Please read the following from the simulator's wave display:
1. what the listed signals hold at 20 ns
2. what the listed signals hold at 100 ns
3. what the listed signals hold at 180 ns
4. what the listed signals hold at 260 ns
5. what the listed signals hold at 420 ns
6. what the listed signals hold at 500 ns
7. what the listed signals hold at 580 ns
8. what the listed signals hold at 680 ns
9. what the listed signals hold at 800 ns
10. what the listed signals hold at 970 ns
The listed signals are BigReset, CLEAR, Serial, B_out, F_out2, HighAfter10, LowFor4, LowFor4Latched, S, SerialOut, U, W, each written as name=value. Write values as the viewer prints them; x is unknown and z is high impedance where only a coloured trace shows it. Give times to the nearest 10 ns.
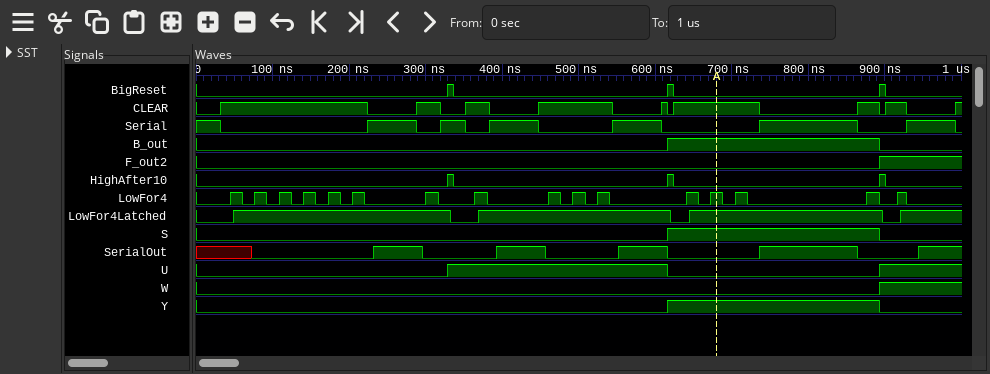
BigReset=0, CLEAR=0, Serial=1, B_out=0, F_out2=0, HighAfter10=0, LowFor4=0, LowFor4Latched=0, S=0, SerialOut=x, U=0, W=0
BigReset=0, CLEAR=1, Serial=0, B_out=0, F_out2=0, HighAfter10=0, LowFor4=0, LowFor4Latched=1, S=0, SerialOut=0, U=0, W=0
BigReset=0, CLEAR=1, Serial=0, B_out=0, F_out2=0, HighAfter10=0, LowFor4=1, LowFor4Latched=1, S=0, SerialOut=0, U=0, W=0
BigReset=0, CLEAR=0, Serial=1, B_out=0, F_out2=0, HighAfter10=0, LowFor4=0, LowFor4Latched=1, S=0, SerialOut=1, U=0, W=0
BigReset=0, CLEAR=0, Serial=1, B_out=0, F_out2=0, HighAfter10=0, LowFor4=0, LowFor4Latched=1, S=0, SerialOut=1, U=1, W=0
BigReset=0, CLEAR=1, Serial=0, B_out=0, F_out2=0, HighAfter10=0, LowFor4=1, LowFor4Latched=1, S=0, SerialOut=0, U=1, W=0
BigReset=0, CLEAR=0, Serial=1, B_out=0, F_out2=0, HighAfter10=0, LowFor4=0, LowFor4Latched=1, S=0, SerialOut=1, U=1, W=0
BigReset=0, CLEAR=1, Serial=0, B_out=1, F_out2=0, HighAfter10=0, LowFor4=1, LowFor4Latched=1, S=1, SerialOut=0, U=0, W=0
BigReset=0, CLEAR=0, Serial=1, B_out=1, F_out2=0, HighAfter10=0, LowFor4=0, LowFor4Latched=1, S=1, SerialOut=1, U=0, W=0
BigReset=0, CLEAR=0, Serial=1, B_out=0, F_out2=1, HighAfter10=0, LowFor4=0, LowFor4Latched=1, S=0, SerialOut=1, U=1, W=1
